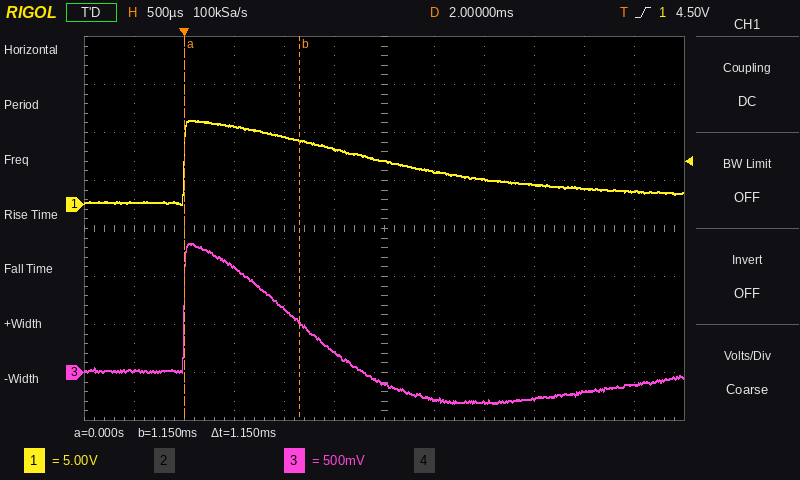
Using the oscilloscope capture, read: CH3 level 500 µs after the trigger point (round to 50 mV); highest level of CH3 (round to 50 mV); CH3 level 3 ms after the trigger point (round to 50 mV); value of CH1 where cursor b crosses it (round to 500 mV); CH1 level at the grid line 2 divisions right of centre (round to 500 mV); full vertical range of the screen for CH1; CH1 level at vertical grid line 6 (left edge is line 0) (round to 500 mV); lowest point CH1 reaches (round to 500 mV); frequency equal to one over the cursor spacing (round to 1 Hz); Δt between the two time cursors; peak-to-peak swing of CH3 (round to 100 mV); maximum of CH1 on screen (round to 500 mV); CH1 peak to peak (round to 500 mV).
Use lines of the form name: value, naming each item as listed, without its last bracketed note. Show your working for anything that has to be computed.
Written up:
CH3 level 500 µs after the trigger point: 1.10 V
highest level of CH3: 1.35 V
CH3 level 3 ms after the trigger point: -300 mV
value of CH1 where cursor b crosses it: 6.5 V
CH1 level at the grid line 2 divisions right of centre: 2.5 V
full vertical range of the screen for CH1: 40 V
CH1 level at vertical grid line 6 (left edge is line 0): 4.5 V
lowest point CH1 reaches: 0.0 V
frequency equal to one over the cursor spacing: 1 / 1.15 ms ≈ 870 Hz
Δt between the two time cursors: 1.15 ms
peak-to-peak swing of CH3: 1.70 V
maximum of CH1 on screen: 9.0 V
CH1 peak to peak: 9.0 V − (0.0 V) = 9.0 V
